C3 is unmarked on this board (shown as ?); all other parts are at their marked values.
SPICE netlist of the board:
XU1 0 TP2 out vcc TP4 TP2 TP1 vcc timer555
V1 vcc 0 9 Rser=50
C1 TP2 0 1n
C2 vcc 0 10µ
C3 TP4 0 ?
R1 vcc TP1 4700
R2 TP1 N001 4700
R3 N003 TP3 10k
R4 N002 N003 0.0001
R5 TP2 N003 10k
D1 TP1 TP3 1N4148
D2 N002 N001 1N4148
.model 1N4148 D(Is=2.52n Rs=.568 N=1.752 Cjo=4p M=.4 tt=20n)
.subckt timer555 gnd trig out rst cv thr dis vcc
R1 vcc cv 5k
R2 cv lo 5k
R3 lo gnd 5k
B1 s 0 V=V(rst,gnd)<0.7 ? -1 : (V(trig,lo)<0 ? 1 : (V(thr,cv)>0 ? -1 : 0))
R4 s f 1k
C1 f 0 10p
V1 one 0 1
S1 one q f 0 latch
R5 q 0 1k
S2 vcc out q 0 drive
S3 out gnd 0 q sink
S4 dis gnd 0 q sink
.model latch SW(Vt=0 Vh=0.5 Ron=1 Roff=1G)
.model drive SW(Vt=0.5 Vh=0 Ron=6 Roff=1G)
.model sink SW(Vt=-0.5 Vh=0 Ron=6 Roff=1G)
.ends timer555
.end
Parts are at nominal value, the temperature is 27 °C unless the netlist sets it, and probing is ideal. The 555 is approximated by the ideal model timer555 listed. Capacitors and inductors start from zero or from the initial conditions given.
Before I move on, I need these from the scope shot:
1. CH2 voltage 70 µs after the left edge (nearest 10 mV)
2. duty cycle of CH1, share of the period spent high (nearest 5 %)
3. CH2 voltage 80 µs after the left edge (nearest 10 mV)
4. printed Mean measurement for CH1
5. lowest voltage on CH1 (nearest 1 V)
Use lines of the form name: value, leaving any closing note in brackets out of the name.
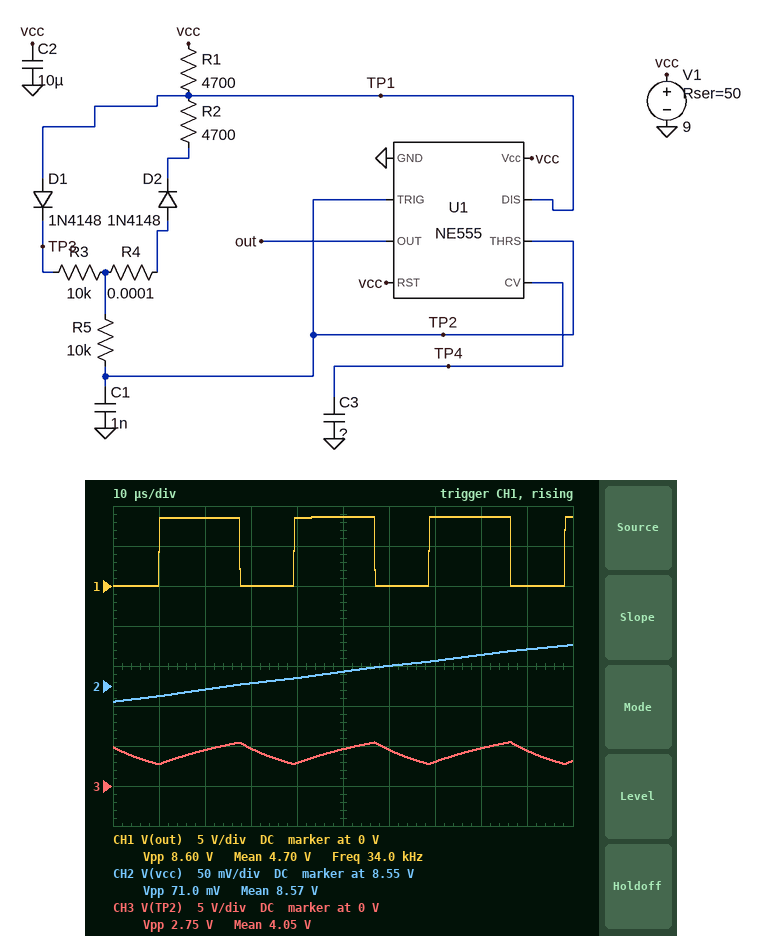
CH2 voltage 70 µs after the left edge: 8.58 V
duty cycle of CH1, share of the period spent high: 60 %
CH2 voltage 80 µs after the left edge: 8.59 V
printed Mean measurement for CH1: 4.70 V
lowest voltage on CH1: 0 V
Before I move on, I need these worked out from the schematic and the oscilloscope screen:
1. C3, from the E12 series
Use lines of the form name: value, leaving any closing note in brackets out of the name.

C3, from the E12 series: 82 nF
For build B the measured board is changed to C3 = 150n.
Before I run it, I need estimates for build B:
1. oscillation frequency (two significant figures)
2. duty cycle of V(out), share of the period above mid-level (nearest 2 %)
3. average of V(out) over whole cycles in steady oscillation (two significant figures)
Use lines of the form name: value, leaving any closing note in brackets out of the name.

oscillation frequency: 37 kHz
duty cycle of V(out), share of the period above mid-level: 56 %
average of V(out) over whole cycles in steady oscillation: 4.8 V
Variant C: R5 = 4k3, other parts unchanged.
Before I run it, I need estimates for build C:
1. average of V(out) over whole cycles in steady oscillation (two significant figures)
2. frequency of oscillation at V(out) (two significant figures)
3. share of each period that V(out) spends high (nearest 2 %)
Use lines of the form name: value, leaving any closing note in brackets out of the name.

average of V(out) over whole cycles in steady oscillation: 5.6 V
frequency of oscillation at V(out): 48 kHz
share of each period that V(out) spends high: 66 %
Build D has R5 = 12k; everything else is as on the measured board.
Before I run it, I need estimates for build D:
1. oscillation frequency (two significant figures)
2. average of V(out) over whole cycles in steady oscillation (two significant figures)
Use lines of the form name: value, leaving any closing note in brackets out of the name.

oscillation frequency: 31 kHz
average of V(out) over whole cycles in steady oscillation: 5.1 V
